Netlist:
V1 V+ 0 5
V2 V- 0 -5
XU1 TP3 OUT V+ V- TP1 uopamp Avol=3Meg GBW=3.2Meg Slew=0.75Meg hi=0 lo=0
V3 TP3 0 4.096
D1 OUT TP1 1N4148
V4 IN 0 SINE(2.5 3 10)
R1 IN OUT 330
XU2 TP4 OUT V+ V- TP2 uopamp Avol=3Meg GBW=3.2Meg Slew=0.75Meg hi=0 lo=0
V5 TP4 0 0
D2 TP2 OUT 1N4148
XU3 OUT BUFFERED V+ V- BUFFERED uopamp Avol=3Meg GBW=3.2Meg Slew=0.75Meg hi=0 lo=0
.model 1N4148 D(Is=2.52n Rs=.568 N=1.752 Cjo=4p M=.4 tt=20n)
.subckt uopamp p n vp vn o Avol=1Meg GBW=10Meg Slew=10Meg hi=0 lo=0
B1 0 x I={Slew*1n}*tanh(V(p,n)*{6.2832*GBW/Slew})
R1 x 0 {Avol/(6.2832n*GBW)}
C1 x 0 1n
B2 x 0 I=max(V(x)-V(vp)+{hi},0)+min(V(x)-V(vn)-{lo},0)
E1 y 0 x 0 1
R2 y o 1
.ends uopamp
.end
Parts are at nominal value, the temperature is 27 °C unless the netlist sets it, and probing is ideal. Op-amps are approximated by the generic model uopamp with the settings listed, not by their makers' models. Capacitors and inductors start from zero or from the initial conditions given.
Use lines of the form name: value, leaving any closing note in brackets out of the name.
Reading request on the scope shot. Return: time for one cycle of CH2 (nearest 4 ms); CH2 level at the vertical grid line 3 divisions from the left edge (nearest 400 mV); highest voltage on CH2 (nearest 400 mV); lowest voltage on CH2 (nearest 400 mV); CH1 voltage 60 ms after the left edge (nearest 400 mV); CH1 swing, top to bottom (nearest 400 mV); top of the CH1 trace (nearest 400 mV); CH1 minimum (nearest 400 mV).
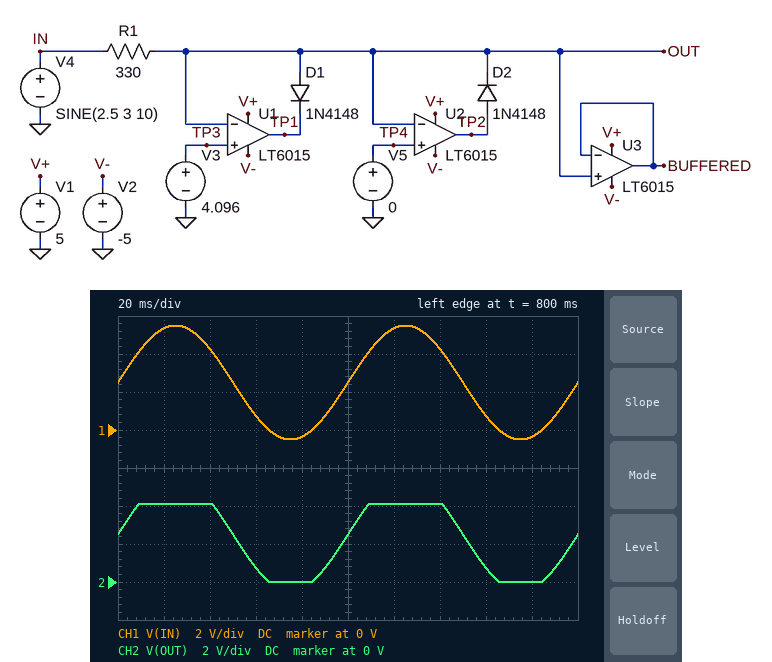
time for one cycle of CH2: 100 ms
CH2 level at the vertical grid line 3 divisions from the left edge: 800 mV
highest voltage on CH2: 4.0 V
lowest voltage on CH2: 0 V
CH1 voltage 60 ms after the left edge: 800 mV
CH1 swing, top to bottom: 6.0 V
top of the CH1 trace: 5.6 V
CH1 minimum: -400 mV
